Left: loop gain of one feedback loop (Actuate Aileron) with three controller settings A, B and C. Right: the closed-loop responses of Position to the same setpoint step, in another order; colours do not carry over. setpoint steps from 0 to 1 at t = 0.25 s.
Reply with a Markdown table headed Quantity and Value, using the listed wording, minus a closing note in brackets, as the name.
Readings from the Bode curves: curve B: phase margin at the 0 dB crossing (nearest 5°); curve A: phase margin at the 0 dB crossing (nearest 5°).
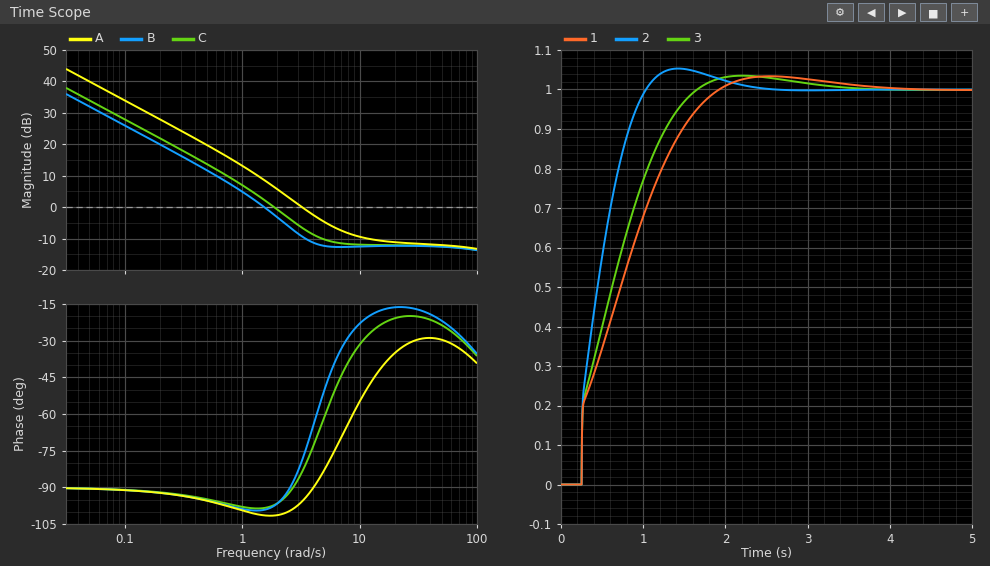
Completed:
| Quantity | Value |
|---|---|
| curve B: phase margin at the 0 dB crossing | 80° |
| curve A: phase margin at the 0 dB crossing | 85° |
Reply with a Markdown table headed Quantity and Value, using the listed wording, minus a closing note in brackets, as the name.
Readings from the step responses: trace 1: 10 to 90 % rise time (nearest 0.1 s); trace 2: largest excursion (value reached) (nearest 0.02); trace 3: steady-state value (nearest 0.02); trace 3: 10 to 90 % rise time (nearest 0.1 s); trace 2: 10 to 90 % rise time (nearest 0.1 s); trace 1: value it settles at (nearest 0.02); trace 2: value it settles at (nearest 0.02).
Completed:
| Quantity | Value |
|---|---|
| trace 1: 10 to 90 % rise time | 1.2 s |
| trace 2: largest excursion (value reached) | 1.06 |
| trace 3: steady-state value | 1.00 |
| trace 3: 10 to 90 % rise time | 1.0 s |
| trace 2: 10 to 90 % rise time | 0.6 s |
| trace 1: value it settles at | 1.00 |
| trace 2: value it settles at | 1.00 |
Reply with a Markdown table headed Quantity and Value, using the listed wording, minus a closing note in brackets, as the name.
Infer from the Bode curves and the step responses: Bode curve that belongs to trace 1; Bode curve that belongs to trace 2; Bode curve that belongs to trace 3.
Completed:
| Quantity | Value |
|---|---|
| Bode curve that belongs to trace 1 | B |
| Bode curve that belongs to trace 2 | A |
| Bode curve that belongs to trace 3 | C |
